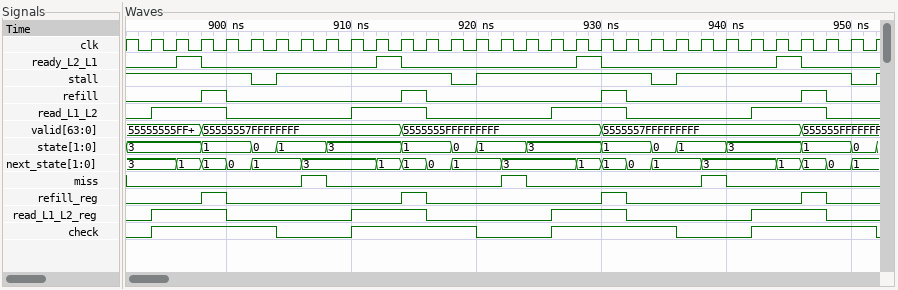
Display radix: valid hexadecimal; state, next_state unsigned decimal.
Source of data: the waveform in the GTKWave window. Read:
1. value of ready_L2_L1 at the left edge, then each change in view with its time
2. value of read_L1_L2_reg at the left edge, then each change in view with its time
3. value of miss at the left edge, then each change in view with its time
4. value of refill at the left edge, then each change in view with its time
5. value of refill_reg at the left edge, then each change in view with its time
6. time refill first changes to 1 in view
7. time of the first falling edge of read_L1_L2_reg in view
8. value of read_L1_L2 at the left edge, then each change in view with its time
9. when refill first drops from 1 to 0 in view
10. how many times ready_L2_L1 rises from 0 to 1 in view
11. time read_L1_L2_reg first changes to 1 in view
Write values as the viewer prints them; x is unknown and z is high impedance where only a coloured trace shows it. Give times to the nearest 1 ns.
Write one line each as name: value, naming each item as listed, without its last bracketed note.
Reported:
value of ready_L2_L1 at the left edge, then each change in view with its time: 0, 1 at 896 ns, 0 at 898 ns, 1 at 912 ns, 0 at 914 ns, 1 at 928 ns, 0 at 930 ns, 1 at 944 ns, 0 at 946 ns
value of read_L1_L2_reg at the left edge, then each change in view with its time: 0, 1 at 894 ns, 0 at 900 ns, 1 at 910 ns, 0 at 916 ns, 1 at 926 ns, 0 at 932 ns, 1 at 942 ns, 0 at 948 ns
value of miss at the left edge, then each change in view with its time: 0, 1 at 906 ns, 0 at 908 ns, 1 at 922 ns, 0 at 924 ns, 1 at 938 ns, 0 at 940 ns
value of refill at the left edge, then each change in view with its time: 0, 1 at 898 ns, 0 at 900 ns, 1 at 914 ns, 0 at 916 ns, 1 at 930 ns, 0 at 932 ns, 1 at 946 ns, 0 at 948 ns
value of refill_reg at the left edge, then each change in view with its time: 0, 1 at 898 ns, 0 at 900 ns, 1 at 914 ns, 0 at 916 ns, 1 at 930 ns, 0 at 932 ns, 1 at 946 ns, 0 at 948 ns
time refill first changes to 1 in view: 898 ns
time of the first falling edge of read_L1_L2_reg in view: 900 ns
value of read_L1_L2 at the left edge, then each change in view with its time: 0, 1 at 894 ns, 0 at 900 ns, 1 at 910 ns, 0 at 916 ns, 1 at 926 ns, 0 at 932 ns, 1 at 942 ns, 0 at 948 ns
when refill first drops from 1 to 0 in view: 900 ns
how many times ready_L2_L1 rises from 0 to 1 in view: 4
time read_L1_L2_reg first changes to 1 in view: 894 ns
